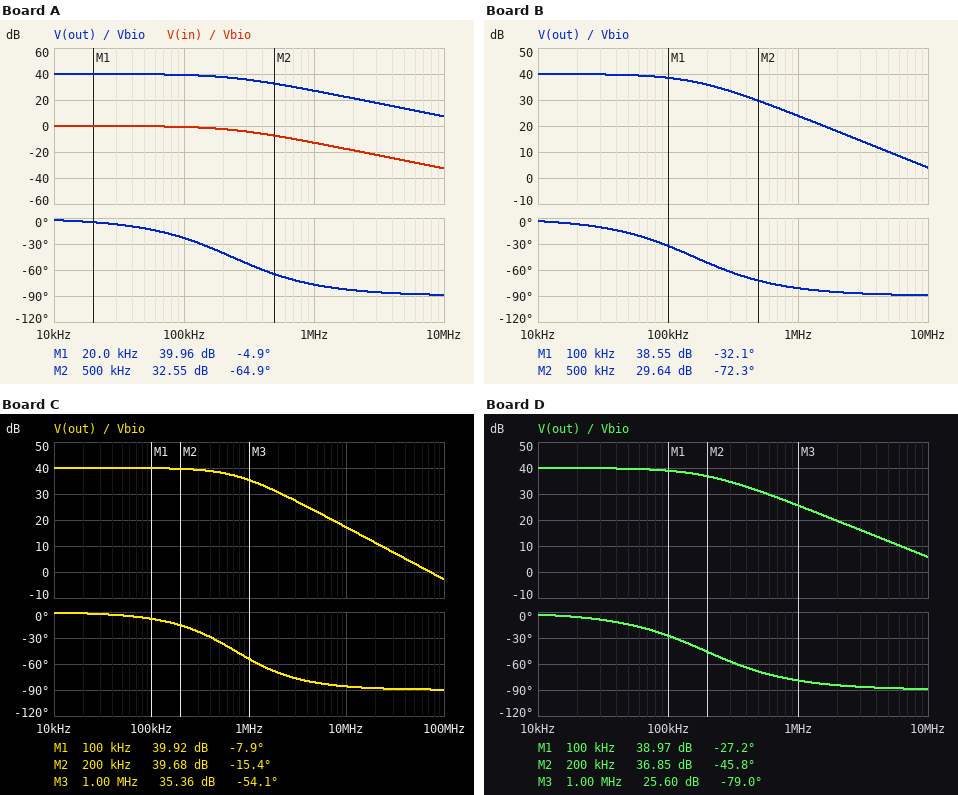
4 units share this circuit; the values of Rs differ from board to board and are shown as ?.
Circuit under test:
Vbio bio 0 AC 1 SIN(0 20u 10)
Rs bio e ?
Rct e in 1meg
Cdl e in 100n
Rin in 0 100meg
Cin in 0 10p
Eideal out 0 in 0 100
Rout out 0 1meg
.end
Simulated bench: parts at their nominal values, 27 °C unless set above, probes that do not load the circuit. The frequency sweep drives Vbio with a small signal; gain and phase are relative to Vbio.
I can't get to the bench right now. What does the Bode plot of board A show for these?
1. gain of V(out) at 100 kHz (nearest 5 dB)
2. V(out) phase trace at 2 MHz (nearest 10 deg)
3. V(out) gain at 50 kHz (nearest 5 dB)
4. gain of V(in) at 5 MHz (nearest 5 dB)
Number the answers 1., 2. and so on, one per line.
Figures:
1. 40 dB
2. -80 deg
3. 40 dB
4. -25 dB
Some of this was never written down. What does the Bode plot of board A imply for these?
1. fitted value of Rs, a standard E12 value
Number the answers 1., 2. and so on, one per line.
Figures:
1. 68 kΩ
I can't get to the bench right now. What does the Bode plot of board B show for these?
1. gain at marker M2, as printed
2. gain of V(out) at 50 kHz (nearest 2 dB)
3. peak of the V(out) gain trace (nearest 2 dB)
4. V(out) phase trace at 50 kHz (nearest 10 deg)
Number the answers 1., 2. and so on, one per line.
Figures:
1. 29.64 dB
2. 40 dB
3. 40 dB
4. -20 deg
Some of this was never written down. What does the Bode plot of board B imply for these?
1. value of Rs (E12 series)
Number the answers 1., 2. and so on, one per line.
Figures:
1. 100 kΩ
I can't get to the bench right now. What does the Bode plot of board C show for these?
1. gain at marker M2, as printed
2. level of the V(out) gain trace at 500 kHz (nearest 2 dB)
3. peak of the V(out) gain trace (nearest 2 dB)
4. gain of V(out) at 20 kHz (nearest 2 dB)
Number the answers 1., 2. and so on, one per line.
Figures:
1. 39.68 dB
2. 38 dB
3. 40 dB
4. 40 dB
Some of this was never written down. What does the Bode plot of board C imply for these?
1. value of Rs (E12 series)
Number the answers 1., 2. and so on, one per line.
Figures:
1. 22 kΩ
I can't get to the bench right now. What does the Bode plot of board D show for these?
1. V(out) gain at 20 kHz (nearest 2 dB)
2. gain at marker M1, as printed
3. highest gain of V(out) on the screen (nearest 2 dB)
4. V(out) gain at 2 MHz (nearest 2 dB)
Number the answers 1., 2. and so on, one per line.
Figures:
1. 40 dB
2. 38.97 dB
3. 40 dB
4. 20 dB
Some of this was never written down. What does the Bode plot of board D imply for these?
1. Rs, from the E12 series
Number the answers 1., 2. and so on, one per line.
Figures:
1. 82 kΩ
